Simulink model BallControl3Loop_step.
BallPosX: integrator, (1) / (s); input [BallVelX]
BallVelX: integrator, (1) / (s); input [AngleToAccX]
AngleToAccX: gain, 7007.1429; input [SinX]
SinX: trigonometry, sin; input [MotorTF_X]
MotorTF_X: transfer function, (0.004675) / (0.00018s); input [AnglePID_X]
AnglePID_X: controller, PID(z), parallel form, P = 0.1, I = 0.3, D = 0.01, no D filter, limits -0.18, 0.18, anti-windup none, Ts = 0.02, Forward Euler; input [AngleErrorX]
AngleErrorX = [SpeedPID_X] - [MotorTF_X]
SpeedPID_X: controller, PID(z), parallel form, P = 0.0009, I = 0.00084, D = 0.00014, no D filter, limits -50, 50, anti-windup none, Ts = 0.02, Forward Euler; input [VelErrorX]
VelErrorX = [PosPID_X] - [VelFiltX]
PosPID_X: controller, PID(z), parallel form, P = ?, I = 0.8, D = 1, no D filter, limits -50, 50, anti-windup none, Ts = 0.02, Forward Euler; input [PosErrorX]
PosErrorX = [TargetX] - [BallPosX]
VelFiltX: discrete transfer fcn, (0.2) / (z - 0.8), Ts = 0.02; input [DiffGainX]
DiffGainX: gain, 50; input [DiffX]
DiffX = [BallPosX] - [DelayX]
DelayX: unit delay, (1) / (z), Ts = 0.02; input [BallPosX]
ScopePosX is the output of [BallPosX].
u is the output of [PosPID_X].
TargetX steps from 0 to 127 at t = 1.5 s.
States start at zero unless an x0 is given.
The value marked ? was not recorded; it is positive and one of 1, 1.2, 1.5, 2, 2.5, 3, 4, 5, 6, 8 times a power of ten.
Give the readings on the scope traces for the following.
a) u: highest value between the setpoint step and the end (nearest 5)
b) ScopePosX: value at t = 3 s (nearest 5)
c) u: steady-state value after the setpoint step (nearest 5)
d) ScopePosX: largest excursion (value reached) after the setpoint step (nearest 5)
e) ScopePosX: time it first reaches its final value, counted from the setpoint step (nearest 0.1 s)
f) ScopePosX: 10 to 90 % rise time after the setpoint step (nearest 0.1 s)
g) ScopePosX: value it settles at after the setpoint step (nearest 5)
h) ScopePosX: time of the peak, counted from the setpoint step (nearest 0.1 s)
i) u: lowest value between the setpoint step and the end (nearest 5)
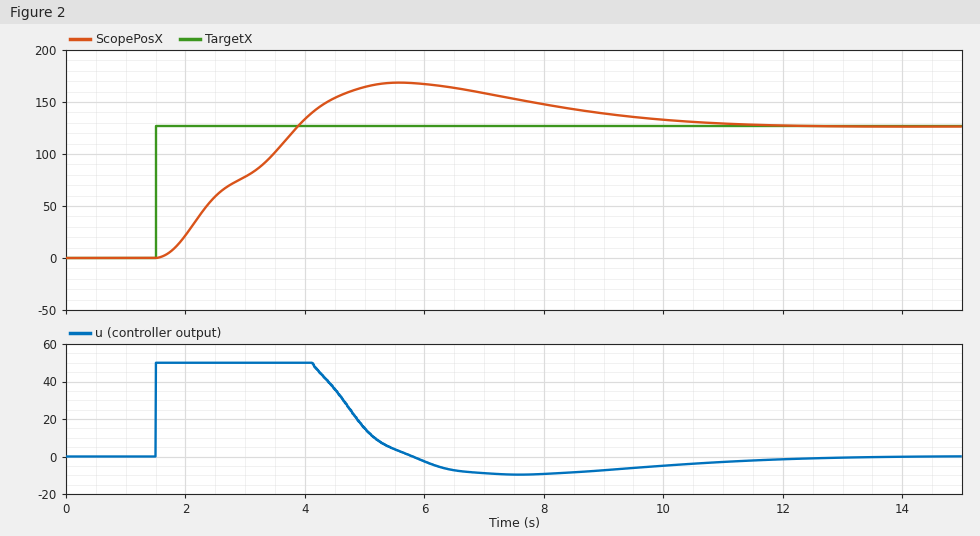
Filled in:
50
80
0
170
2.4 s
1.8 s
125
4.1 s
-10
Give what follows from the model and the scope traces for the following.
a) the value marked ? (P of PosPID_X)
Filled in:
2
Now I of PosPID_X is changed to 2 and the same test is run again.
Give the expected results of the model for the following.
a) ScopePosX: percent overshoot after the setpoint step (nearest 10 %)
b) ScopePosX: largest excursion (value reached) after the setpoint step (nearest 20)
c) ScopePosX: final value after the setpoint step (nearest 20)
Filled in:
60 %
200
120
